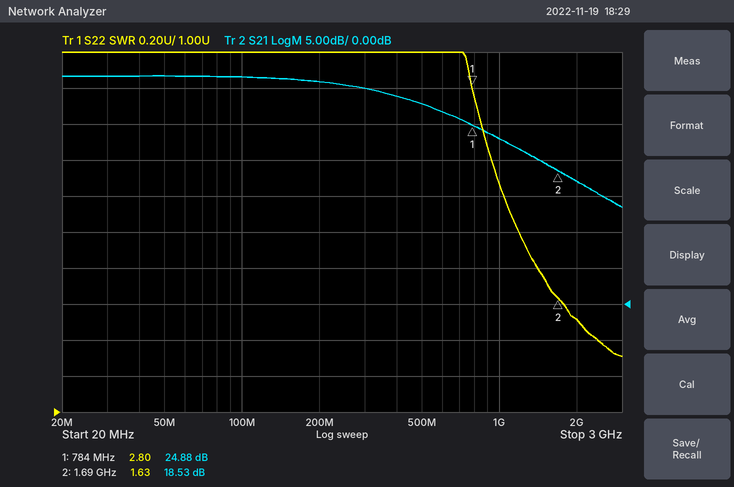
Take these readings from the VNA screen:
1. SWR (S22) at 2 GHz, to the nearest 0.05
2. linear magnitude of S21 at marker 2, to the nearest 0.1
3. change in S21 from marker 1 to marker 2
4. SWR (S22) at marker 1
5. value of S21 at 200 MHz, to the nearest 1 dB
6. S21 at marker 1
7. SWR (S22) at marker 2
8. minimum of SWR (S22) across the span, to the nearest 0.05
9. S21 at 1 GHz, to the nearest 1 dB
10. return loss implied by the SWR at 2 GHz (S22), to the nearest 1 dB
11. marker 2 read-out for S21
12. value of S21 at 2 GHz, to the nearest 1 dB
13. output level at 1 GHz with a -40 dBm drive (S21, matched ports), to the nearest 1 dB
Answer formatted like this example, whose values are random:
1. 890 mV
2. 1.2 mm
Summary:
1. 1.50
2. 8.4
3. -6.35 dB
4. 2.80
5. 31 dB
6. 24.88 dB
7. 1.63
8. 1.30
9. 23 dB
10. 14 dB
11. 18.53 dB
12. 17 dB
13. -17 dBm
